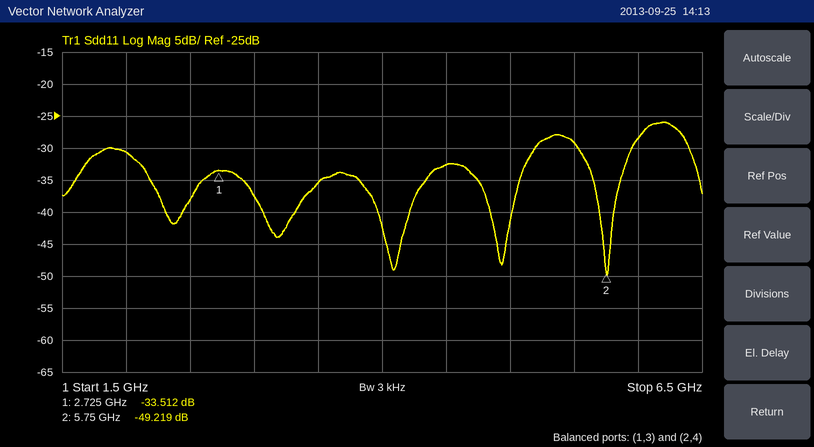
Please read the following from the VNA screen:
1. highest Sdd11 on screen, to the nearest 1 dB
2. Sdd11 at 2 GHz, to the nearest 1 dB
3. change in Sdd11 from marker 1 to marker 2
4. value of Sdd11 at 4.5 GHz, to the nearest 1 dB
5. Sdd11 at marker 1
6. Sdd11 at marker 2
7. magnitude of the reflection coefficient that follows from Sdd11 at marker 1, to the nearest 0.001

-26 dB
-31 dB
-15.707 dB
-33 dB
-33.512 dB
-49.219 dB
0.021
